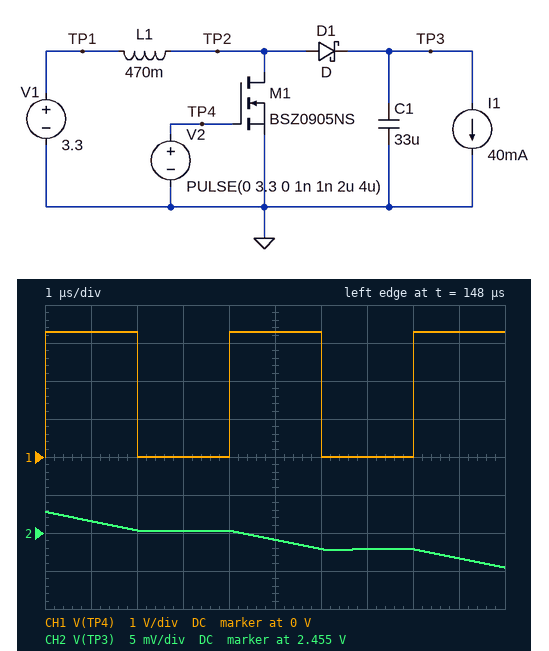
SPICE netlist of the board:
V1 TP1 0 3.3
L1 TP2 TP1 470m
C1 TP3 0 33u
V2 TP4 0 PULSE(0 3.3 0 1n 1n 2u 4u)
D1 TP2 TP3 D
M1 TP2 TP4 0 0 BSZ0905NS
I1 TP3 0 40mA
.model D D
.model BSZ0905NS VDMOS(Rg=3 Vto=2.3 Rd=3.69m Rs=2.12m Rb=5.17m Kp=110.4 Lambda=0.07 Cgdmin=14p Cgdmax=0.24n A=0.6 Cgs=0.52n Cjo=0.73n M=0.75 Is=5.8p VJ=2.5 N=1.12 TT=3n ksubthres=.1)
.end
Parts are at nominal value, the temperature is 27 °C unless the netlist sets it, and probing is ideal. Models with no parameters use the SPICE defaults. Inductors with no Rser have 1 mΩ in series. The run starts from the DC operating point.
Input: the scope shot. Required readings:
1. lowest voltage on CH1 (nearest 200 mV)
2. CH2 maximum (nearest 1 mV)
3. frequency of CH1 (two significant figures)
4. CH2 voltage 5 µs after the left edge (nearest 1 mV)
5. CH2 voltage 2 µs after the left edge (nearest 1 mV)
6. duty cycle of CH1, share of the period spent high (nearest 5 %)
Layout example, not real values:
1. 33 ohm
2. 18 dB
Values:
1. 0 V
2. 2.458 V
3. 250 kHz
4. 2.454 V
5. 2.455 V
6. 50 %
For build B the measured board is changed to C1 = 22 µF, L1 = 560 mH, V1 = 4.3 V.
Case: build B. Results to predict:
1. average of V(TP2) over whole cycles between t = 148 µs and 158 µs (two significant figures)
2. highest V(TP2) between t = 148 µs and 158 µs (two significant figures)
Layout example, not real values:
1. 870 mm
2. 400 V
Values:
1. 2.0 V
2. 4.2 V
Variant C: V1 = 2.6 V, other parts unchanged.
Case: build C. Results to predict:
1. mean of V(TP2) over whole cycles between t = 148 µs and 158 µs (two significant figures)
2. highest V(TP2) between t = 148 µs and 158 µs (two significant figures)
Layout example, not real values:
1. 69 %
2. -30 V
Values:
1. 1.2 V
2. 2.5 V
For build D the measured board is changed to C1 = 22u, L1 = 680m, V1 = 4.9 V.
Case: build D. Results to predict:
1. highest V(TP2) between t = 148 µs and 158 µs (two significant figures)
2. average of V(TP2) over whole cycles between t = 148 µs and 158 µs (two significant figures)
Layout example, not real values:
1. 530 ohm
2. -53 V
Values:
1. 4.8 V
2. 2.3 V
